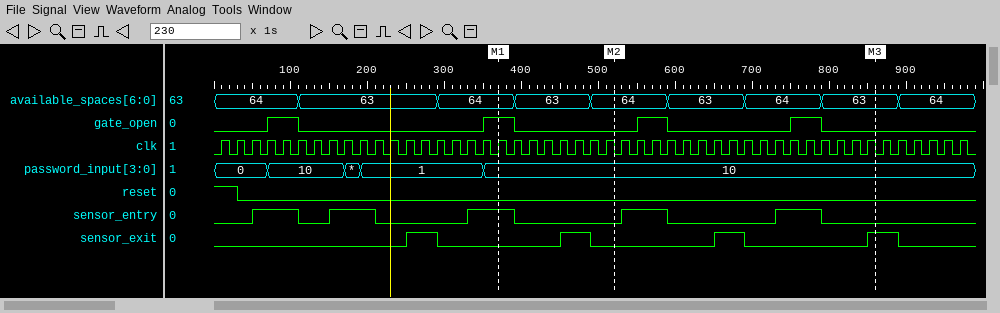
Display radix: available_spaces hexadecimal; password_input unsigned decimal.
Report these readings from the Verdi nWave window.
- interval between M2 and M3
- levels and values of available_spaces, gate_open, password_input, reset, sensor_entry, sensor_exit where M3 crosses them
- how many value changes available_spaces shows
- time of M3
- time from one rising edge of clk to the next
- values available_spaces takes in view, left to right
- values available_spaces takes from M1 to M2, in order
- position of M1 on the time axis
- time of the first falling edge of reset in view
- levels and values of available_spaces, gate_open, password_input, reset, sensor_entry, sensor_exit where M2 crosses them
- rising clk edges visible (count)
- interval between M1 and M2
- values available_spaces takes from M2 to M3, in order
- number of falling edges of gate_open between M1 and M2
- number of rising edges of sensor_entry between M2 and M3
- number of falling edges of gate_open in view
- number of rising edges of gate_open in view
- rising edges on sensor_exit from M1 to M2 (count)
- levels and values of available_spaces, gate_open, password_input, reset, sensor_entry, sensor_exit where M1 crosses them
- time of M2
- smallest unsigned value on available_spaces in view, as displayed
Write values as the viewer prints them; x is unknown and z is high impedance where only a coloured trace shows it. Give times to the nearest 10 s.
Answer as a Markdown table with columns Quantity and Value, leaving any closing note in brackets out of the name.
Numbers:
| Quantity | Value |
|---|---|
| interval between M2 and M3 | 340 s |
| levels and values of available_spaces, gate_open, password_input, reset, sensor_entry, sensor_exit where M3 crosses them | available_spaces=63, gate_open=0, password_input=10, reset=0, sensor_entry=0, sensor_exit=1 |
| how many value changes available_spaces shows | 8 |
| time of M3 | 860 s |
| time from one rising edge of clk to the next | 20 s |
| values available_spaces takes in view, left to right | 64, 63, 64, 63, 64, 63, 64, 63, 64 |
| values available_spaces takes from M1 to M2, in order | 64, 63, 64 |
| position of M1 on the time axis | 370 s |
| time of the first falling edge of reset in view | 30 s |
| levels and values of available_spaces, gate_open, password_input, reset, sensor_entry, sensor_exit where M2 crosses them | available_spaces=64, gate_open=0, password_input=10, reset=0, sensor_entry=0, sensor_exit=0 |
| rising clk edges visible | 49 |
| interval between M1 and M2 | 150 s |
| values available_spaces takes from M2 to M3, in order | 64, 63, 64, 63 |
| number of falling edges of gate_open between M1 and M2 | 1 |
| number of rising edges of sensor_entry between M2 and M3 | 2 |
| number of falling edges of gate_open in view | 4 |
| number of rising edges of gate_open in view | 4 |
| rising edges on sensor_exit from M1 to M2 | 1 |
| levels and values of available_spaces, gate_open, password_input, reset, sensor_entry, sensor_exit where M1 crosses them | available_spaces=64, gate_open=1, password_input=10, reset=0, sensor_entry=1, sensor_exit=0 |
| time of M2 | 520 s |
| smallest unsigned value on available_spaces in view, as displayed | 63 |
